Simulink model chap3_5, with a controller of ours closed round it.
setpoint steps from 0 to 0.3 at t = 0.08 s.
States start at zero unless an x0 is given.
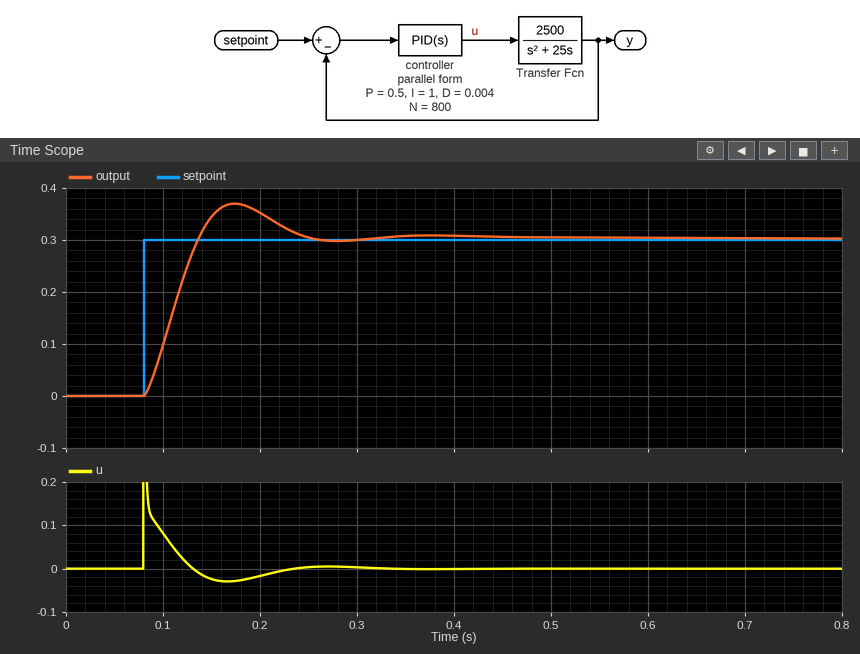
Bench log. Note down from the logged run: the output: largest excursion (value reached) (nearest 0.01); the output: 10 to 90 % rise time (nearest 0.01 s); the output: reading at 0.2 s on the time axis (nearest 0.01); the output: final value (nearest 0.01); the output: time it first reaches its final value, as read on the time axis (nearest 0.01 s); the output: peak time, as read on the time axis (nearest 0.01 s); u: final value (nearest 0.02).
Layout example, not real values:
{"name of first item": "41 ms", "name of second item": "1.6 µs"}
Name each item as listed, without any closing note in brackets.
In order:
{"the output: largest excursion (value reached)": "0.37", "the output: 10 to 90 % rise time": "0.04 s", "the output: reading at 0.2 s on the time axis": "0.35", "the output: final value": "0.30", "the output: time it first reaches its final value, as read on the time axis": "0.14 s", "the output: peak time, as read on the time axis": "0.17 s", "u: final value": "0.00"}
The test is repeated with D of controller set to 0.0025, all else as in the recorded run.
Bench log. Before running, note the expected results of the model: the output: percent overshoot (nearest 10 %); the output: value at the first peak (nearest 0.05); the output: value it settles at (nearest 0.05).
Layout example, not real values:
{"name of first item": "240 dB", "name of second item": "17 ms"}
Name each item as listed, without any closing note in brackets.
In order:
{"the output: percent overshoot": "30 %", "the output: value at the first peak": "0.40", "the output: value it settles at": "0.30"}
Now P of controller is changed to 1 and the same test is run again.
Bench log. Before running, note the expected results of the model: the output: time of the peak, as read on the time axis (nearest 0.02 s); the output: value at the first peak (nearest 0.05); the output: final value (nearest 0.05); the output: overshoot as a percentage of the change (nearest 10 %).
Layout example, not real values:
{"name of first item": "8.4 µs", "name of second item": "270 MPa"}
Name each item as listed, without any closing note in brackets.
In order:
{"the output: time of the peak, as read on the time axis": "0.14 s", "the output: value at the first peak": "0.40", "the output: final value": "0.30", "the output: overshoot as a percentage of the change": "30 %"}
